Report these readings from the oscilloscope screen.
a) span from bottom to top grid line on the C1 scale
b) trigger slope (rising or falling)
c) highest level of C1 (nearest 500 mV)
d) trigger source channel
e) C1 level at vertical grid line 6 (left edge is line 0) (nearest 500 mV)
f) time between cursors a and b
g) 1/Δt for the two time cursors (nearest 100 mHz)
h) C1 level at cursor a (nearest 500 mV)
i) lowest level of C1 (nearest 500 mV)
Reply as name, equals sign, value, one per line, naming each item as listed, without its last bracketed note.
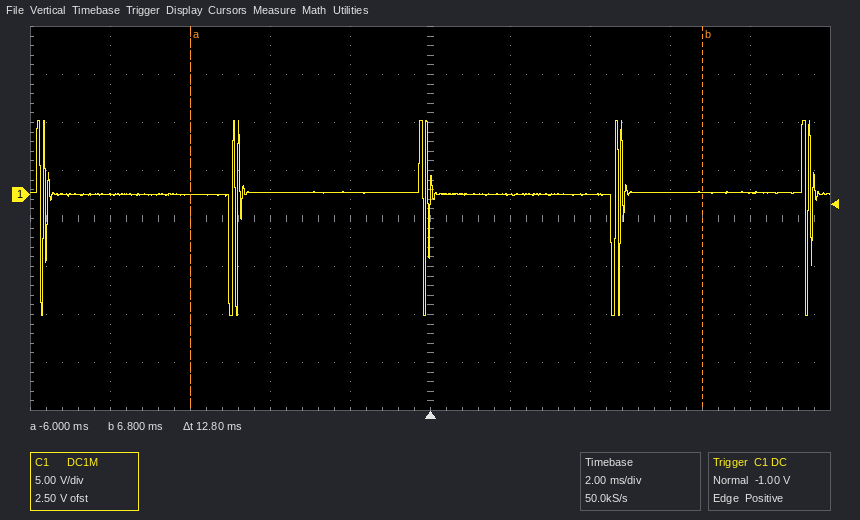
span from bottom to top grid line on the C1 scale = 40 V
trigger slope = rising
highest level of C1 = 7.5 V
trigger source channel = C1
C1 level at vertical grid line 6 (left edge is line 0) = 0.0 V
time between cursors a and b = 12.8 ms
1/Δt for the two time cursors = 78.1 Hz
C1 level at cursor a = 0.0 V
lowest level of C1 = -12.5 V
